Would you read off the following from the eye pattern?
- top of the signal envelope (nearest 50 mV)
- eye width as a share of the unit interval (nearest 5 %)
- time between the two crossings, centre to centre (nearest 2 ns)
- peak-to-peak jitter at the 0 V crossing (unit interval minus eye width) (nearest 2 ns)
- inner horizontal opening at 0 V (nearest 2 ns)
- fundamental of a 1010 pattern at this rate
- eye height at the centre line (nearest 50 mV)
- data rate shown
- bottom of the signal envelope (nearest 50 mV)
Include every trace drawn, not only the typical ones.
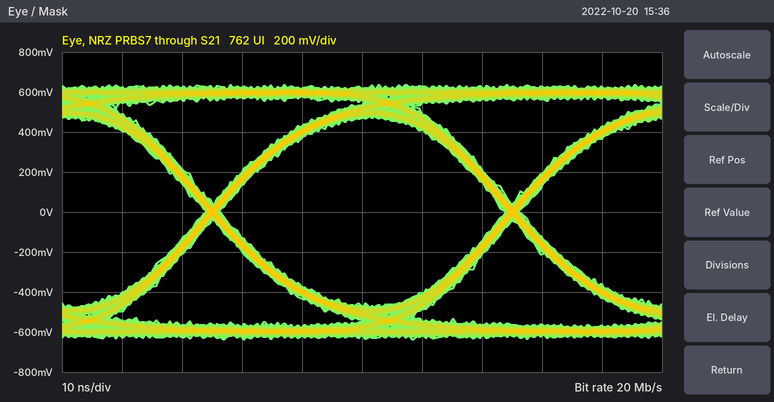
650 mV
95 %
50 ns
2 ns
48 ns
10 MHz
950 mV
20 Mb/s
-650 mV
